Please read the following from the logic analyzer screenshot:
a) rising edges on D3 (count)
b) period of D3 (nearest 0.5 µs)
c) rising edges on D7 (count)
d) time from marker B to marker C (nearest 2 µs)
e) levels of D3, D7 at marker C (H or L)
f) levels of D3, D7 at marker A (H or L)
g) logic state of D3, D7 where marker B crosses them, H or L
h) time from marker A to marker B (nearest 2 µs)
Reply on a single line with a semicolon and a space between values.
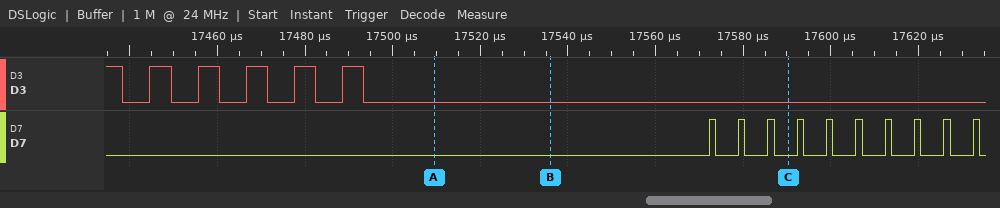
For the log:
5; 11 µs; 10; 54 µs; D3=L, D7=L; D3=L, D7=L; D3=L, D7=L; 26 µs
